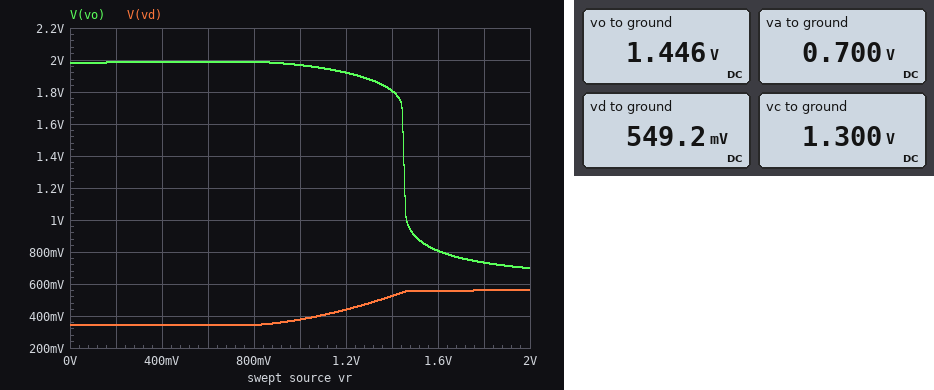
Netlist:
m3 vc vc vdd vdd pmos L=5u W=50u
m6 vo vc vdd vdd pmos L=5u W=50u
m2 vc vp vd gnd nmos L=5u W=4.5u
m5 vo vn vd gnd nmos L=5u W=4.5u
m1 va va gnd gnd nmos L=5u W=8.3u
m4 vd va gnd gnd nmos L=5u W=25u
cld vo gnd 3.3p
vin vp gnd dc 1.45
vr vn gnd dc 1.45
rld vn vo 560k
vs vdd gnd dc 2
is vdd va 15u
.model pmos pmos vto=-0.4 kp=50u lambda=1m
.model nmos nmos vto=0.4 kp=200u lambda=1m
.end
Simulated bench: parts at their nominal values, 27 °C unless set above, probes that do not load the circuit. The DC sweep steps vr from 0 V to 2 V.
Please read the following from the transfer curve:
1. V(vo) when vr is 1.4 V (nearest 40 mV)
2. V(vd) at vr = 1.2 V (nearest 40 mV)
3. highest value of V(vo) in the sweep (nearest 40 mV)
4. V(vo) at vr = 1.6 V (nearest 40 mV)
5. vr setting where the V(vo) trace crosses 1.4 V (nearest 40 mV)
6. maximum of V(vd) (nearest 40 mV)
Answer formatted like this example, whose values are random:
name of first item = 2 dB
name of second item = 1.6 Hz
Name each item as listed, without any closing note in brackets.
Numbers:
V(vo) when vr is 1.4 V = 1.80 V
V(vd) at vr = 1.2 V = 440 mV
highest value of V(vo) in the sweep = 2.00 V
V(vo) at vr = 1.6 V = 800 mV
vr setting where the V(vo) trace crosses 1.4 V = 1.44 V
maximum of V(vd) = 560 mV
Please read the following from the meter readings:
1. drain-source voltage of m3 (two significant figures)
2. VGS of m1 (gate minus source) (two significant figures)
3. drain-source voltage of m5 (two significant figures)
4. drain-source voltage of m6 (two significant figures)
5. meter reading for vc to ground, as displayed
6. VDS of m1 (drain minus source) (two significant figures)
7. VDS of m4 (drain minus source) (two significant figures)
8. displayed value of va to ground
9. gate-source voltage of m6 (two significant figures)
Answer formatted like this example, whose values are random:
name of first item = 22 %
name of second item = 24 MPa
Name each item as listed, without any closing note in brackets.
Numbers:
drain-source voltage of m3 = -700 mV
VGS of m1 (gate minus source) = 700 mV
drain-source voltage of m5 = 900 mV
drain-source voltage of m6 = -550 mV
meter reading for vc to ground, as displayed = 1.300 V
VDS of m1 (drain minus source) = 700 mV
VDS of m4 (drain minus source) = 550 mV
displayed value of va to ground = 0.700 V
gate-source voltage of m6 = -700 mV
